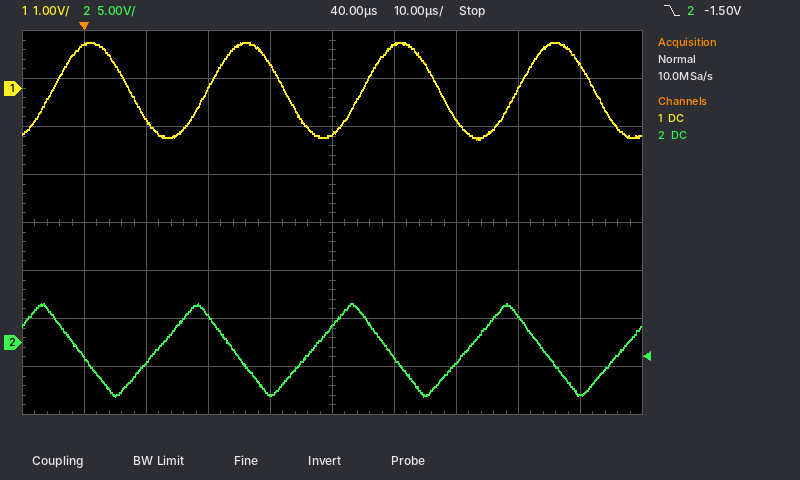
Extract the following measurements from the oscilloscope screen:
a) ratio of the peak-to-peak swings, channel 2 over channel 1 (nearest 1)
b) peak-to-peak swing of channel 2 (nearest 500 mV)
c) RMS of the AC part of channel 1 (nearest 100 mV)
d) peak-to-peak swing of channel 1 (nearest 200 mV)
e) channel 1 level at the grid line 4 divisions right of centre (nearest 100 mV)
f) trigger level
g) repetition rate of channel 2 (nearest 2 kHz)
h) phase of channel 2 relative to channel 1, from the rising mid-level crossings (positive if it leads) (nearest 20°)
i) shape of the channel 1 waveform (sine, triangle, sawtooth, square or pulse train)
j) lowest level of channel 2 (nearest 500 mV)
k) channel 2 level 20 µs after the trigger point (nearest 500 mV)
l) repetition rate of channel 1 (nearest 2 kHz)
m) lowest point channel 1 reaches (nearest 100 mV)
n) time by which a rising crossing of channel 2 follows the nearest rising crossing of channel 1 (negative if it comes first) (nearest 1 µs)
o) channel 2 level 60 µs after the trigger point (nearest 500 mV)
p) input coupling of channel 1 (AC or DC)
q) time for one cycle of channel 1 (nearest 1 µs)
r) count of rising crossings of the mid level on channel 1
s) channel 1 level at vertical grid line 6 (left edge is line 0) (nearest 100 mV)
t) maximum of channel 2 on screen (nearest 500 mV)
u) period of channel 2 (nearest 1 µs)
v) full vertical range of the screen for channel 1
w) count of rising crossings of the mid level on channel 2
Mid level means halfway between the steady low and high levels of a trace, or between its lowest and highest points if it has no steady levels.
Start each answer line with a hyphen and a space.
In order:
- 5
- 9.5 V
- 700 mV
- 2.0 V
- 500 mV
- -1.50 V
- 40 kHz
- +120°
- sine
- -5.5 V
- 3.0 V
- 40 kHz
- -1.1 V
- -8 µs
- -2.0 V
- DC
- 25 µs
- 4
- 900 mV
- 4.0 V
- 25 µs
- 8 V
- 4
